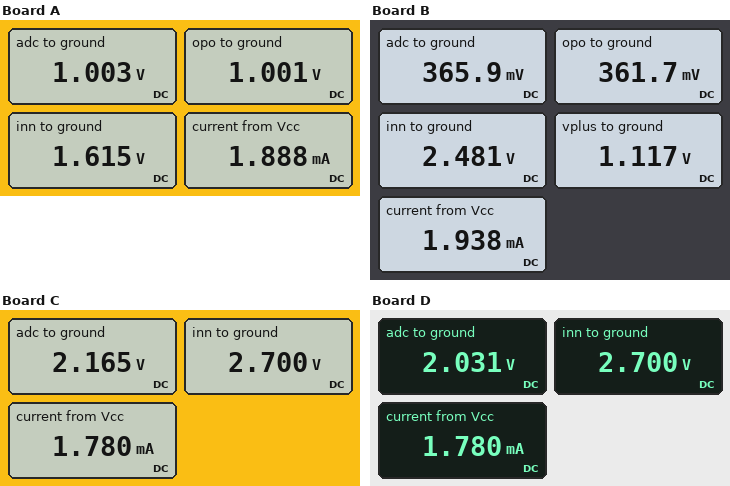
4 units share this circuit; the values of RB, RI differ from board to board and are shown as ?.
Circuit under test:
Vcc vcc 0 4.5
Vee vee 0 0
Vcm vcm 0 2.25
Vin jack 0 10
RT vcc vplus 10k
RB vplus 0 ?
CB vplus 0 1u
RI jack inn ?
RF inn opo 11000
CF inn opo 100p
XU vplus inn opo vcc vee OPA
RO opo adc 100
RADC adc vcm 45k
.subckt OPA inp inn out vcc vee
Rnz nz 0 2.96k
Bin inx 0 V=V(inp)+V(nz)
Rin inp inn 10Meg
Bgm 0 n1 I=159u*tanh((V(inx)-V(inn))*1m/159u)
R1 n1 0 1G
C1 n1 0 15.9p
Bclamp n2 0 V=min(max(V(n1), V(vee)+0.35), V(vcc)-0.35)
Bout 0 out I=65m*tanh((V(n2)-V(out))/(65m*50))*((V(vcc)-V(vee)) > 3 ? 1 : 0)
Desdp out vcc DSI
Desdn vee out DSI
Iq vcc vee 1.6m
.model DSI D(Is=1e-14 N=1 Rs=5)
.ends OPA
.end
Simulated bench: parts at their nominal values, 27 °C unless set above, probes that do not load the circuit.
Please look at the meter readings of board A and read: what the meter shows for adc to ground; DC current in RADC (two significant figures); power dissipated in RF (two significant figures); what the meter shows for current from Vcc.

1.003 V
28 µA
34 µW
1.888 mA
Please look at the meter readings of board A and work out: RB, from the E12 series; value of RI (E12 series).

5.6 kΩ
150 kΩ
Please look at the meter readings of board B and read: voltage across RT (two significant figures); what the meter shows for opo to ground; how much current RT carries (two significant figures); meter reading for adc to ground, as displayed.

3.4 V
361.7 mV
340 µA
365.9 mV
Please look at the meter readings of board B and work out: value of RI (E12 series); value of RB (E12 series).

39 kΩ
3.3 kΩ
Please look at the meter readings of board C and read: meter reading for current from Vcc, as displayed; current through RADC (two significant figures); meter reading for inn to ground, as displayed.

1.780 mA
1.9 µA
2.700 V
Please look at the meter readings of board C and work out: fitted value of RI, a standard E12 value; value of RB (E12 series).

150 kΩ
15 kΩ
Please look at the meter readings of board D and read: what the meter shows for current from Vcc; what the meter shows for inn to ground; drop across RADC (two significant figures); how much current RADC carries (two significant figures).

1.780 mA
2.700 V
220 mV
4.9 µA
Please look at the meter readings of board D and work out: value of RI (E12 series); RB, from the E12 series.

120 kΩ
15 kΩ
